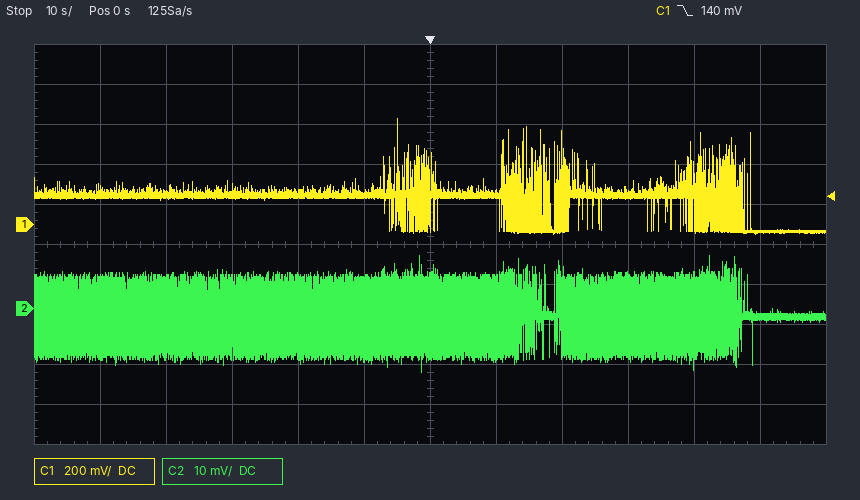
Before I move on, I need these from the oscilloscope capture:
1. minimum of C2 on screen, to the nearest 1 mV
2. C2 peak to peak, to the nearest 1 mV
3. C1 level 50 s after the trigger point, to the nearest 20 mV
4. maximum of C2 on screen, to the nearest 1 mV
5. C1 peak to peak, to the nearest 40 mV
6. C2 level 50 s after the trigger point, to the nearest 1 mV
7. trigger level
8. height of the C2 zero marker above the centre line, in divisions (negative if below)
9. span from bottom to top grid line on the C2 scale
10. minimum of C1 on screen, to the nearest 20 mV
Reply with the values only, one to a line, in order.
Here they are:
-16 mV
29 mV
-40 mV
13 mV
560 mV
-2 mV
140 mV
-1.6 div
100 mV
-40 mV
